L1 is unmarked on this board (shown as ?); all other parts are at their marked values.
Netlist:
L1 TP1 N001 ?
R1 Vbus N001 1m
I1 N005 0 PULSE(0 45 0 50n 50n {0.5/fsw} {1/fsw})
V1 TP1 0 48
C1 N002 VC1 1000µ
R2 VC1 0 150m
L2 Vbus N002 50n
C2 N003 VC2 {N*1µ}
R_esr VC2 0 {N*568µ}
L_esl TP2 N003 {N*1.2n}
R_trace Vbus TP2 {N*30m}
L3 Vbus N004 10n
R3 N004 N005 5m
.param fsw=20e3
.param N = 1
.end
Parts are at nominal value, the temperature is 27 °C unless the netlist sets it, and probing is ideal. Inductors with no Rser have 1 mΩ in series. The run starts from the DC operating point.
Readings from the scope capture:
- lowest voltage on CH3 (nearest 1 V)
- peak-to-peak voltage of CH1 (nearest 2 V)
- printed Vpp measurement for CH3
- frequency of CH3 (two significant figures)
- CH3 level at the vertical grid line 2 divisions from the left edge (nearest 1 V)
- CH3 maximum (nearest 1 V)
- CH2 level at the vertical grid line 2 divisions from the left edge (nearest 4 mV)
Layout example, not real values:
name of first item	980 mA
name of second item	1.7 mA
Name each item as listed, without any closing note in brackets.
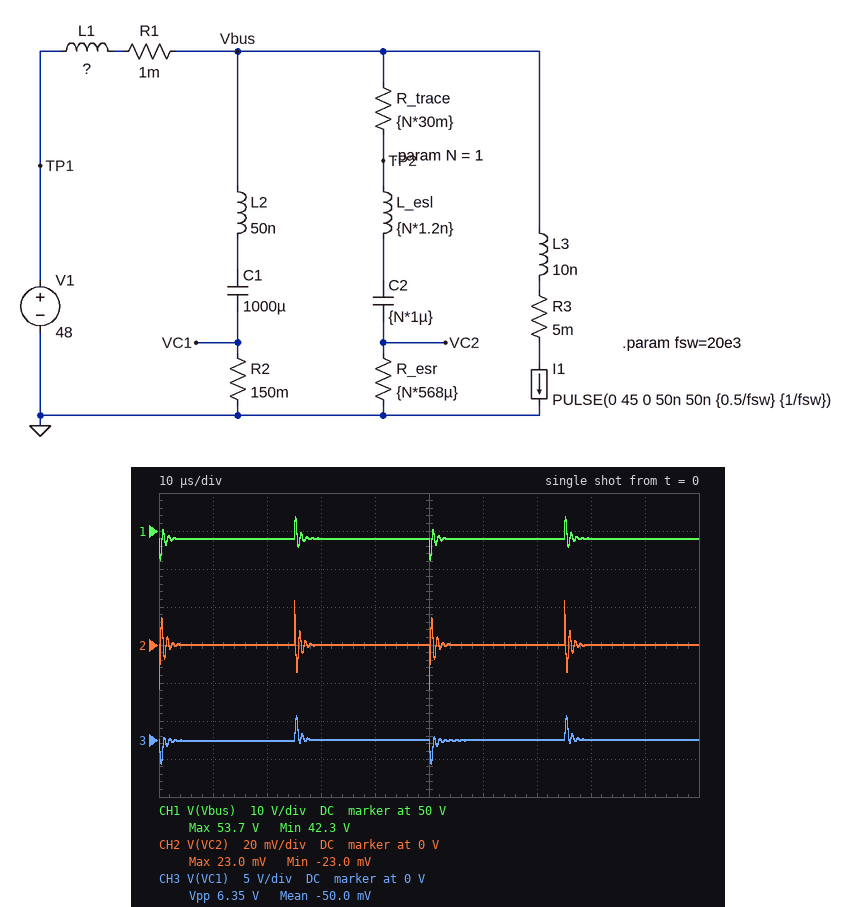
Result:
lowest voltage on CH3	-3 V
peak-to-peak voltage of CH1	12 V
printed Vpp measurement for CH3	6.35 V
frequency of CH3	20 kHz
CH3 level at the vertical grid line 2 divisions from the left edge	0 V
CH3 maximum	3 V
CH2 level at the vertical grid line 2 divisions from the left edge	0 V
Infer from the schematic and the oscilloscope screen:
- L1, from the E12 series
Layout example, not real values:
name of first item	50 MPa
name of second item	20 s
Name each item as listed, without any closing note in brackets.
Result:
L1, from the E12 series	39 nH
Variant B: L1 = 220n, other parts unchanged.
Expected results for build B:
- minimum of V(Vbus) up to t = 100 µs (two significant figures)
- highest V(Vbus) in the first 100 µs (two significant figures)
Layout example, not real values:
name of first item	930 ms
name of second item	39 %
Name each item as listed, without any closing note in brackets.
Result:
minimum of V(Vbus) up to t = 100 µs	39 V
highest V(Vbus) in the first 100 µs	57 V
